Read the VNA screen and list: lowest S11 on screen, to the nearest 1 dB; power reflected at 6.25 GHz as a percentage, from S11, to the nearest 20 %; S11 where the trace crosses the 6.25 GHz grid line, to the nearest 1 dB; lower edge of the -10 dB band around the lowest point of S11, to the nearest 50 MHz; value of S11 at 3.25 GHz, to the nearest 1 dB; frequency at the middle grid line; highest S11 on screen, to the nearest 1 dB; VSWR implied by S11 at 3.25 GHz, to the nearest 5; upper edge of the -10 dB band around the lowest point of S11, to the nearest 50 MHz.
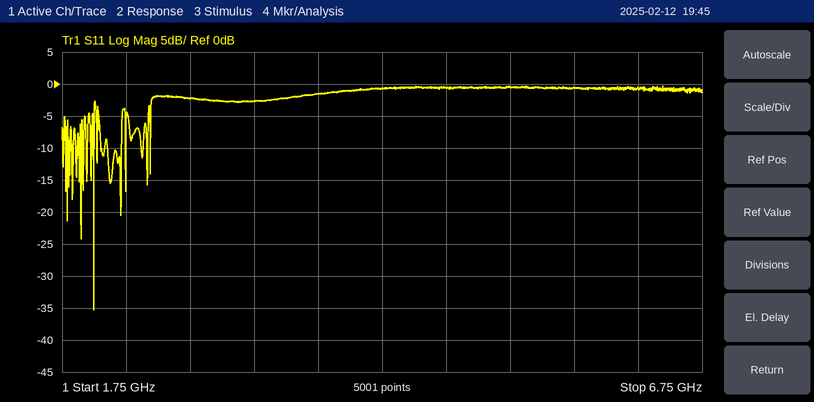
-35 dB
80 %
-1 dB
2.00 GHz
-3 dB
4.25 GHz
0 dB
5
2.00 GHz
